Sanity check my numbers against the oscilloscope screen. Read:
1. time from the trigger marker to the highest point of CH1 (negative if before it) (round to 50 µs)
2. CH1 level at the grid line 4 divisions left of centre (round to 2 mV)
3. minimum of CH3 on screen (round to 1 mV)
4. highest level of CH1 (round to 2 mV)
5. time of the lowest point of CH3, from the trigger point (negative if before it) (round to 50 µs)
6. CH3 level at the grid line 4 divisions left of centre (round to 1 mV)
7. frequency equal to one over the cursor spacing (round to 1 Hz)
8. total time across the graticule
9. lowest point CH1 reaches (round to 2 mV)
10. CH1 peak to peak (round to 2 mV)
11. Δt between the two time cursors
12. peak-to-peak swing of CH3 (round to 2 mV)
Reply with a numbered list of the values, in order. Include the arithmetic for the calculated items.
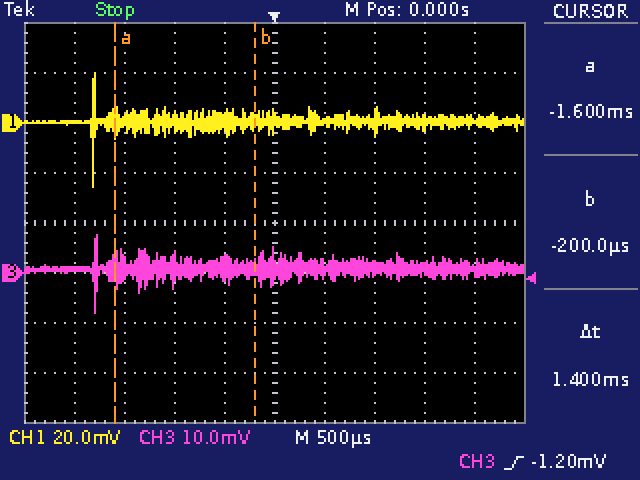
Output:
1. -1.80 ms
2. 0 mV
3. -8 mV
4. 20 mV
5. -1.80 ms
6. 1 mV
7. 1 / 1.4 ms ≈ 714 Hz
8. 5 ms
9. -26 mV
10. 20 mV − (-26 mV) = 46 mV
11. 1.4 ms
12. 16 mV
